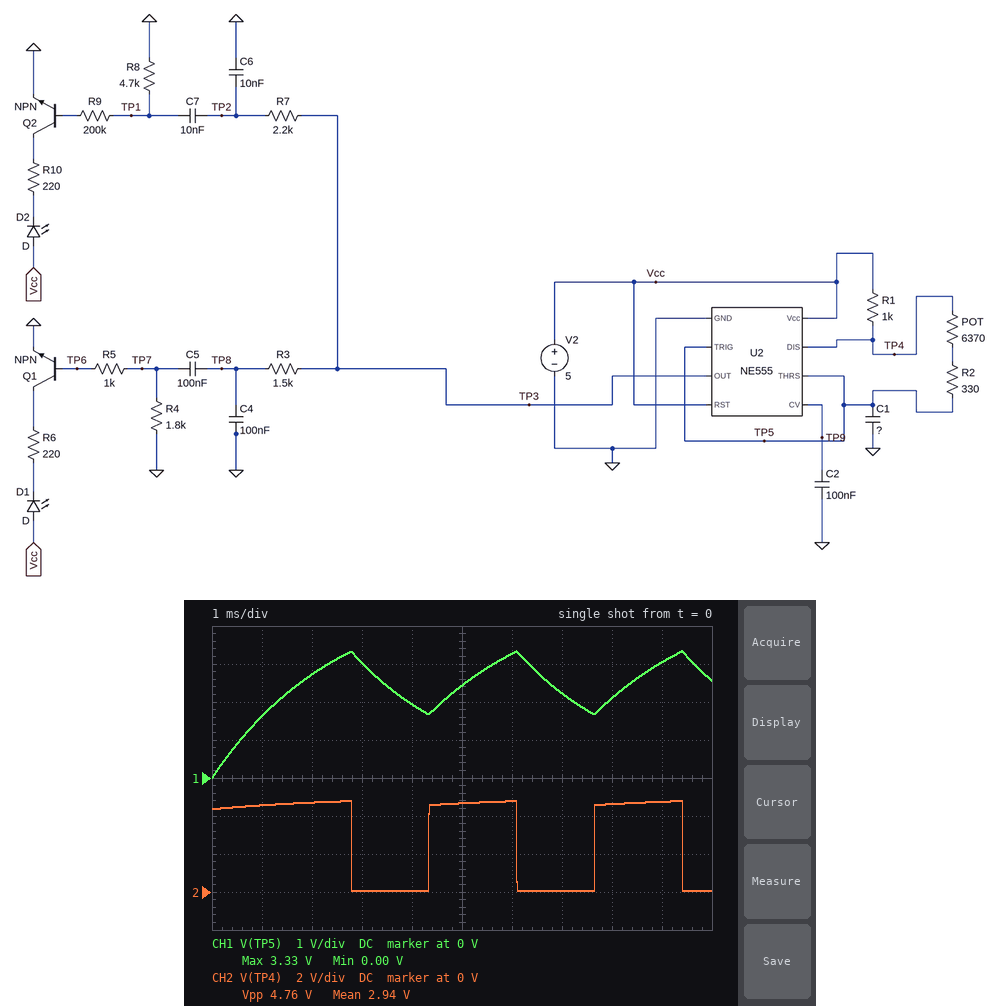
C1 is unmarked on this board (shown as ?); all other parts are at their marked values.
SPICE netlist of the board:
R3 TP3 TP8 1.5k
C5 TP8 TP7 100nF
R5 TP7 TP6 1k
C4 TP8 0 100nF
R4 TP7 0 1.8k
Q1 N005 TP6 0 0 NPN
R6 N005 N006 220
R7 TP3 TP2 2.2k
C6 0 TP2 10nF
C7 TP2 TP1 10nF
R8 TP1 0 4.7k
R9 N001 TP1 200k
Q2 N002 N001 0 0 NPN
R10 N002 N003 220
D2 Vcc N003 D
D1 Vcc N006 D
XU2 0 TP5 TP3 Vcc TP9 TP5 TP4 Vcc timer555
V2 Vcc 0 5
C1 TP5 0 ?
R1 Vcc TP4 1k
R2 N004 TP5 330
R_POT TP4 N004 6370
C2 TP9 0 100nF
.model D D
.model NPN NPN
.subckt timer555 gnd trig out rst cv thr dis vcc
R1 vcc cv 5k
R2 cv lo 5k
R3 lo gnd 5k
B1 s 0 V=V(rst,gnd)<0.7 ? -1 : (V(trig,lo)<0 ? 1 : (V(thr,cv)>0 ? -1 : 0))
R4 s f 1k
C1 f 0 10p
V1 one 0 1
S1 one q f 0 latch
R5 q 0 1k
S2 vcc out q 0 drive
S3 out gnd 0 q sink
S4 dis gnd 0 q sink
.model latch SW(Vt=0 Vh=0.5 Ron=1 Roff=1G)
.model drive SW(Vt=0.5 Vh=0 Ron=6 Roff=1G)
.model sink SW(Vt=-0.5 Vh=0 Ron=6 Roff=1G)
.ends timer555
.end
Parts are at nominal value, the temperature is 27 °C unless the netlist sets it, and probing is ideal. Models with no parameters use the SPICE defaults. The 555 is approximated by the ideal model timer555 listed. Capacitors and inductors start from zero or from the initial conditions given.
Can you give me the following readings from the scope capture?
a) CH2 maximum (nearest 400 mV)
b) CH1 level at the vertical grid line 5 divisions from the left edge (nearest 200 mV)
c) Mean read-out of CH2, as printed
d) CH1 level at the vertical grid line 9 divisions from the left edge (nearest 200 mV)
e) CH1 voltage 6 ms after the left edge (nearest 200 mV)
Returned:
4.8 V
2.4 V
2.94 V
3.0 V
3.2 V
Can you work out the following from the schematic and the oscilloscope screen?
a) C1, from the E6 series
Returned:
330 nF
